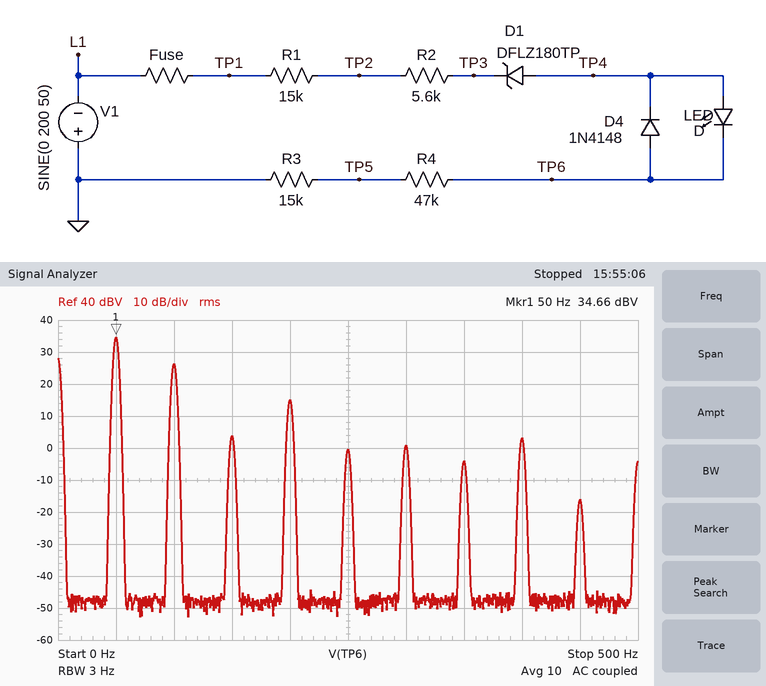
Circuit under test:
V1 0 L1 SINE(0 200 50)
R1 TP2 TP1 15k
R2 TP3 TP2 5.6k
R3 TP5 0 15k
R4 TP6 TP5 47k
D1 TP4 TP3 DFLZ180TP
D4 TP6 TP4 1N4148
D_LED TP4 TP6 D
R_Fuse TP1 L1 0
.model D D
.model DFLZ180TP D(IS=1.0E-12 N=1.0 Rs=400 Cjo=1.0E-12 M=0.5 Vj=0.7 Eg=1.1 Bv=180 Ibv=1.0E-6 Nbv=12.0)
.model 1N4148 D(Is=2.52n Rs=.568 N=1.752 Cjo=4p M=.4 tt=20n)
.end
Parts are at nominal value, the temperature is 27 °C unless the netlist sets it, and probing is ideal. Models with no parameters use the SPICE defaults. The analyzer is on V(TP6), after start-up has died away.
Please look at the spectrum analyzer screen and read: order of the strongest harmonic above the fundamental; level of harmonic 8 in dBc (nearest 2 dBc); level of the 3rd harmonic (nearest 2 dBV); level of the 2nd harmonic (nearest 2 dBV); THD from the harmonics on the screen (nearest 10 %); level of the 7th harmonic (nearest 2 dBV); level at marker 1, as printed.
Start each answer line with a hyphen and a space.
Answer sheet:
- 2
- -32 dBc
- 4 dBV
- 26 dBV
- 40 %
- -4 dBV
- 34.66 dBV
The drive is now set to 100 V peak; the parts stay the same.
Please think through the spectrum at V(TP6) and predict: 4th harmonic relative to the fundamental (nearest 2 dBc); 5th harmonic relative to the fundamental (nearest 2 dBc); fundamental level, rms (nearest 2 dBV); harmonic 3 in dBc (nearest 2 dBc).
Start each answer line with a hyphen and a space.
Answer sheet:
- -22 dBc
- -52 dBc
- 28 dBV
- -48 dBc
